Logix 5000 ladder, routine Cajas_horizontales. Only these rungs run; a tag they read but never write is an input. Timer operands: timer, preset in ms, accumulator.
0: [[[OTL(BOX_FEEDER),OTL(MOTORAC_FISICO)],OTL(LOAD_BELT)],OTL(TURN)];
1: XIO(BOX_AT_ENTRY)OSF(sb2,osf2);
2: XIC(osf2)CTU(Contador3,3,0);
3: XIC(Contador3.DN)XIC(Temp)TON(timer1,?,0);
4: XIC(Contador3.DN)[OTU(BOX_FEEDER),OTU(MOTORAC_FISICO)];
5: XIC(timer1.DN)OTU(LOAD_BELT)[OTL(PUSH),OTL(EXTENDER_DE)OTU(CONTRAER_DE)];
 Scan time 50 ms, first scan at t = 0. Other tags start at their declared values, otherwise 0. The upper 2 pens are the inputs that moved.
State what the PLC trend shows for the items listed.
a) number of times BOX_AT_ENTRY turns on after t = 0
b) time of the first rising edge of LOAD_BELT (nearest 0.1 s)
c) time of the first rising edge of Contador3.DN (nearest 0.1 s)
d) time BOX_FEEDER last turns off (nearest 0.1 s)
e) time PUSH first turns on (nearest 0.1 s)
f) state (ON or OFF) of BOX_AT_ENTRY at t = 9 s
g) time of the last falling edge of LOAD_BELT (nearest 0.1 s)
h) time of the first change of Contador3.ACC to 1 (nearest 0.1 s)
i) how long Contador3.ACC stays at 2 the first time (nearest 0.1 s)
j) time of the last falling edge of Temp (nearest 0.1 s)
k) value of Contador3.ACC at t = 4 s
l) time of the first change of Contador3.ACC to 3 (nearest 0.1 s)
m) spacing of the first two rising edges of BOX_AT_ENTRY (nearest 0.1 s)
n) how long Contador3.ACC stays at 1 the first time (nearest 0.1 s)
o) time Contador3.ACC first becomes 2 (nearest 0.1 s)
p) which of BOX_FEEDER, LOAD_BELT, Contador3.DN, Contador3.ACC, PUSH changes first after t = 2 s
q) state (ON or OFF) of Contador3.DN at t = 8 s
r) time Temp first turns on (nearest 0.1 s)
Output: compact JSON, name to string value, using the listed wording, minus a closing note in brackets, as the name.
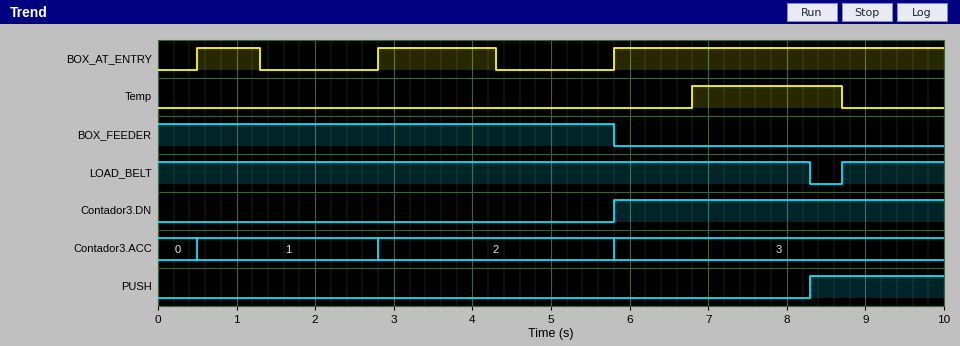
{"number of times BOX_AT_ENTRY turns on after t = 0": "3", "time of the first rising edge of LOAD_BELT": "8.7 s", "time of the first rising edge of Contador3.DN": "5.8 s", "time BOX_FEEDER last turns off": "5.8 s", "time PUSH first turns on": "8.3 s", "state (ON or OFF) of BOX_AT_ENTRY at t = 9 s": "ON", "time of the last falling edge of LOAD_BELT": "8.3 s", "time of the first change of Contador3.ACC to 1": "0.5 s", "how long Contador3.ACC stays at 2 the first time": "3.0 s", "time of the last falling edge of Temp": "8.7 s", "value of Contador3.ACC at t = 4 s": "2", "time of the first change of Contador3.ACC to 3": "5.8 s", "spacing of the first two rising edges of BOX_AT_ENTRY": "2.3 s", "how long Contador3.ACC stays at 1 the first time": "2.3 s", "time Contador3.ACC first becomes 2": "2.8 s", "which of BOX_FEEDER, LOAD_BELT, Contador3.DN, Contador3.ACC, PUSH changes first after t = 2 s": "Contador3.ACC", "state (ON or OFF) of Contador3.DN at t = 8 s": "ON", "time Temp first turns on": "6.8 s"}
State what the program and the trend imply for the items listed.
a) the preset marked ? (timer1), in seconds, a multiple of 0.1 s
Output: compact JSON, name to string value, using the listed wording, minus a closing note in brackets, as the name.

{"the preset marked ? (timer1), in seconds, a multiple of 0.1 s": "1.5 s"}
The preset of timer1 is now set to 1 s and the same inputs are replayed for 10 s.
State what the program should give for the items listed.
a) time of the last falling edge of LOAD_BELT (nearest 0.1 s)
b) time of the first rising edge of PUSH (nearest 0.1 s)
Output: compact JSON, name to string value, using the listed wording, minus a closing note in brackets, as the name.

{"time of the last falling edge of LOAD_BELT": "7.8 s", "time of the first rising edge of PUSH": "7.8 s"}
